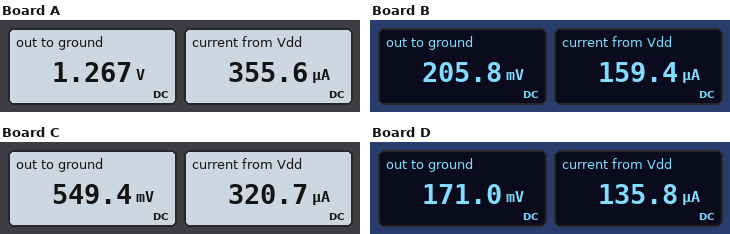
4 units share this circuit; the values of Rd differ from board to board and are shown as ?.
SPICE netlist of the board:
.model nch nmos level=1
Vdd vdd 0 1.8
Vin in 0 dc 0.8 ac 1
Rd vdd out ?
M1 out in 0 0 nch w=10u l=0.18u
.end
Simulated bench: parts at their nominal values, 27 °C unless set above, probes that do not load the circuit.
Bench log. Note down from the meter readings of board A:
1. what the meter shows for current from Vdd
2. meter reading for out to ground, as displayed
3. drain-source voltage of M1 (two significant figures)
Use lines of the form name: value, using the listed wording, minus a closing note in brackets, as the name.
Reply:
what the meter shows for current from Vdd: 355.6 µA
meter reading for out to ground, as displayed: 1.267 V
drain-source voltage of M1: 1.3 V
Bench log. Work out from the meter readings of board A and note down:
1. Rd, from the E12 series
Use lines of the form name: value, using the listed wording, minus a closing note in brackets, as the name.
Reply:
Rd, from the E12 series: 1.5 kΩ
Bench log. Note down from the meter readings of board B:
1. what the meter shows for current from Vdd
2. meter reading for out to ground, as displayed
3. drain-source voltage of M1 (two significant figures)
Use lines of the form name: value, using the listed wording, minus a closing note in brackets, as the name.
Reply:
what the meter shows for current from Vdd: 159.4 µA
meter reading for out to ground, as displayed: 205.8 mV
drain-source voltage of M1: 210 mV
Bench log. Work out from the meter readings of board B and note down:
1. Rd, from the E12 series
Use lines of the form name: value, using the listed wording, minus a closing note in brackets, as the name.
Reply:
Rd, from the E12 series: 10 kΩ
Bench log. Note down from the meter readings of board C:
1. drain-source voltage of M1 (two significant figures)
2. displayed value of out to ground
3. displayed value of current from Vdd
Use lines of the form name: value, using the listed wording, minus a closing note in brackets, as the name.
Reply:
drain-source voltage of M1: 550 mV
displayed value of out to ground: 549.4 mV
displayed value of current from Vdd: 320.7 µA
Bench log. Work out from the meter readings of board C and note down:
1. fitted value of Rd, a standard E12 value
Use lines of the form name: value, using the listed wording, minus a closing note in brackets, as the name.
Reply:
fitted value of Rd, a standard E12 value: 3.9 kΩ
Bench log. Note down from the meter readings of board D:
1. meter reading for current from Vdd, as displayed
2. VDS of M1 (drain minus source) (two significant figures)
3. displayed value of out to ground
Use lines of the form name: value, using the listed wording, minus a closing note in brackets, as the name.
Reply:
meter reading for current from Vdd, as displayed: 135.8 µA
VDS of M1 (drain minus source): 170 mV
displayed value of out to ground: 171.0 mV
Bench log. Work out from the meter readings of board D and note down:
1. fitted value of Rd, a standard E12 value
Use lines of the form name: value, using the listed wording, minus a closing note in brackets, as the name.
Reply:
fitted value of Rd, a standard E12 value: 12 kΩ
